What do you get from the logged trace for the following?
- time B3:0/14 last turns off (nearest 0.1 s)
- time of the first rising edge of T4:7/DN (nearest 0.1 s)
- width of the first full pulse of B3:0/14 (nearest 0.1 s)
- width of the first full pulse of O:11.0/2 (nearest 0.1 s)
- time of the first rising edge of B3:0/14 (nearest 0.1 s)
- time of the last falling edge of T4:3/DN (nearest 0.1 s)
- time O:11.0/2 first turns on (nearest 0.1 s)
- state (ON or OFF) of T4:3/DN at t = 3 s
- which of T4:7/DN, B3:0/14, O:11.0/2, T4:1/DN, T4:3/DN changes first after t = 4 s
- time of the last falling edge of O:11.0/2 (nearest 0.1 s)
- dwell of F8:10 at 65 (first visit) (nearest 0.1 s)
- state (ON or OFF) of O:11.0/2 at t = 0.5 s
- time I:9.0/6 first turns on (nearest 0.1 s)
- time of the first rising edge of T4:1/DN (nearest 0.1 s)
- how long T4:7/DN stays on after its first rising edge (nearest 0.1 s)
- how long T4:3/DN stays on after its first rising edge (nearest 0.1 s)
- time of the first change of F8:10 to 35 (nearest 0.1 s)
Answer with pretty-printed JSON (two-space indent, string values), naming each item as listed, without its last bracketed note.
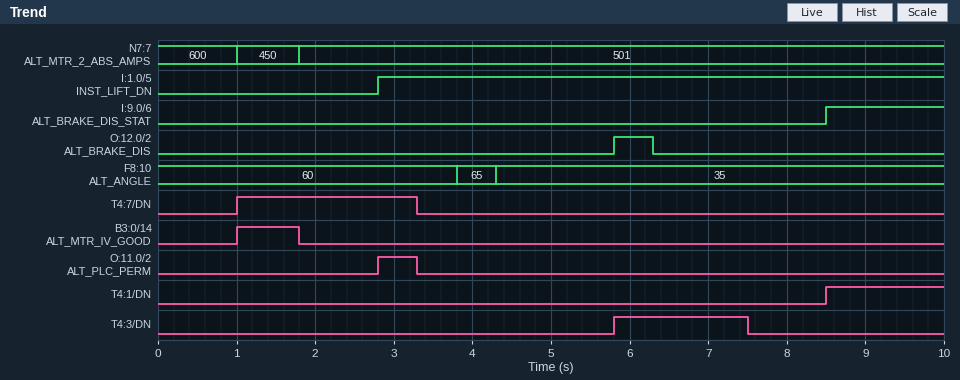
{
  "time B3:0/14 last turns off": "1.8 s",
  "time of the first rising edge of T4:7/DN": "1.0 s",
  "width of the first full pulse of B3:0/14": "0.8 s",
  "width of the first full pulse of O:11.0/2": "0.5 s",
  "time of the first rising edge of B3:0/14": "1.0 s",
  "time of the last falling edge of T4:3/DN": "7.5 s",
  "time O:11.0/2 first turns on": "2.8 s",
  "state (ON or OFF) of T4:3/DN at t = 3 s": "OFF",
  "which of T4:7/DN, B3:0/14, O:11.0/2, T4:1/DN, T4:3/DN changes first after t = 4 s": "T4:3/DN",
  "time of the last falling edge of O:11.0/2": "3.3 s",
  "dwell of F8:10 at 65 (first visit)": "0.5 s",
  "state (ON or OFF) of O:11.0/2 at t = 0.5 s": "OFF",
  "time I:9.0/6 first turns on": "8.5 s",
  "time of the first rising edge of T4:1/DN": "8.5 s",
  "how long T4:7/DN stays on after its first rising edge": "2.3 s",
  "how long T4:3/DN stays on after its first rising edge": "1.7 s",
  "time of the first change of F8:10 to 35": "4.3 s"
}
